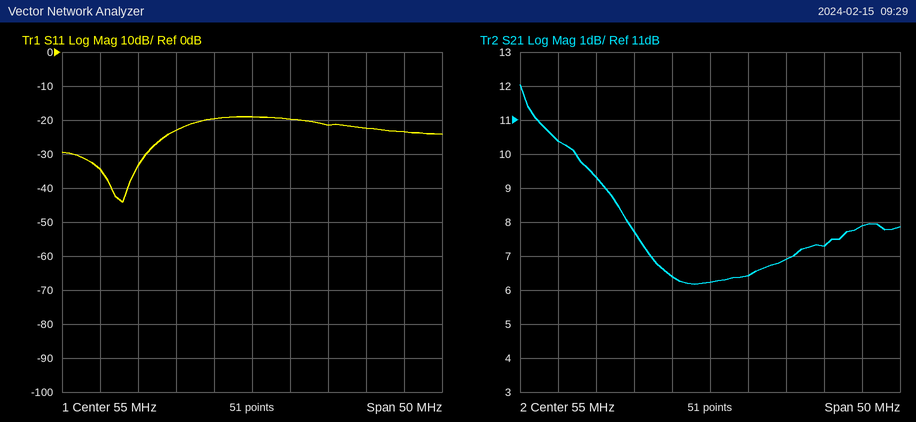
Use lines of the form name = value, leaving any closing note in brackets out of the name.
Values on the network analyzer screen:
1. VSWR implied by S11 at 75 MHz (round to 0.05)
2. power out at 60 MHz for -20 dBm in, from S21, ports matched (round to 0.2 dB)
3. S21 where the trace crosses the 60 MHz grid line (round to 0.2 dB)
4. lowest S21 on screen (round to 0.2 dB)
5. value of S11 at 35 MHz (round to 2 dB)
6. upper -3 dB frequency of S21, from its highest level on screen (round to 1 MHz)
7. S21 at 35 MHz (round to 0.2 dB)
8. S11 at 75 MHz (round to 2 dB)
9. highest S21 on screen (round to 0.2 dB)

VSWR implied by S11 at 75 MHz = 1.15
power out at 60 MHz for -20 dBm in, from S21, ports matched = -13.6 dBm
S21 where the trace crosses the 60 MHz grid line = 6.4 dB
lowest S21 on screen = 6.2 dB
value of S11 at 35 MHz = -34 dB
upper -3 dB frequency of S21, from its highest level on screen = 41 MHz
S21 at 35 MHz = 10.4 dB
S11 at 75 MHz = -24 dB
highest S21 on screen = 12.0 dB
